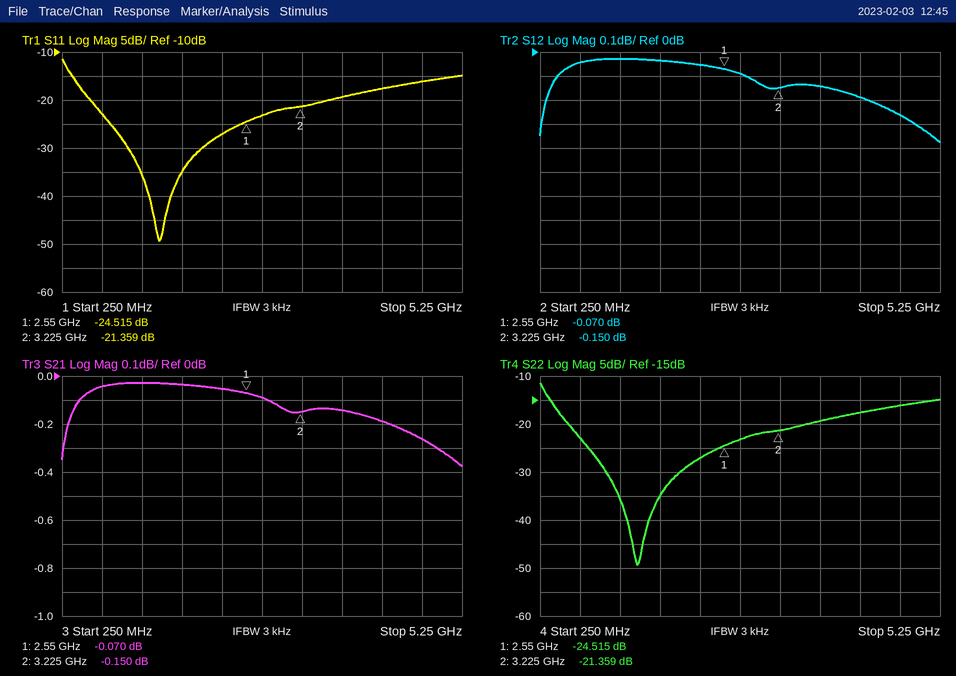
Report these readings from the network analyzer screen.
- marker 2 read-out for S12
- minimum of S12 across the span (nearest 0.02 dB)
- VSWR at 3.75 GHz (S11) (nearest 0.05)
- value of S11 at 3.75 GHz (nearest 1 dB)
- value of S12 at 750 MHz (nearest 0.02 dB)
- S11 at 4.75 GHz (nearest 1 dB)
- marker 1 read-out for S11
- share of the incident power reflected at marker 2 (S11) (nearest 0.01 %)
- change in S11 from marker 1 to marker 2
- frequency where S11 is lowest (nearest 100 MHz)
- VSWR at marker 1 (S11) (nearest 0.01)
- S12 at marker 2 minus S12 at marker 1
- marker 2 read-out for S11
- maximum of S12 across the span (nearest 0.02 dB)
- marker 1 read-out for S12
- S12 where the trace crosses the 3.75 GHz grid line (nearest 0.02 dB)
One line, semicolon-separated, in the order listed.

-0.150 dB; -0.38 dB; 1.25; -19 dB; -0.04 dB; -16 dB; -24.515 dB; 0.73 %; 3.156 dB; 1.5 GHz; 1.13; -0.080 dB; -21.359 dB; -0.02 dB; -0.070 dB; -0.14 dB
